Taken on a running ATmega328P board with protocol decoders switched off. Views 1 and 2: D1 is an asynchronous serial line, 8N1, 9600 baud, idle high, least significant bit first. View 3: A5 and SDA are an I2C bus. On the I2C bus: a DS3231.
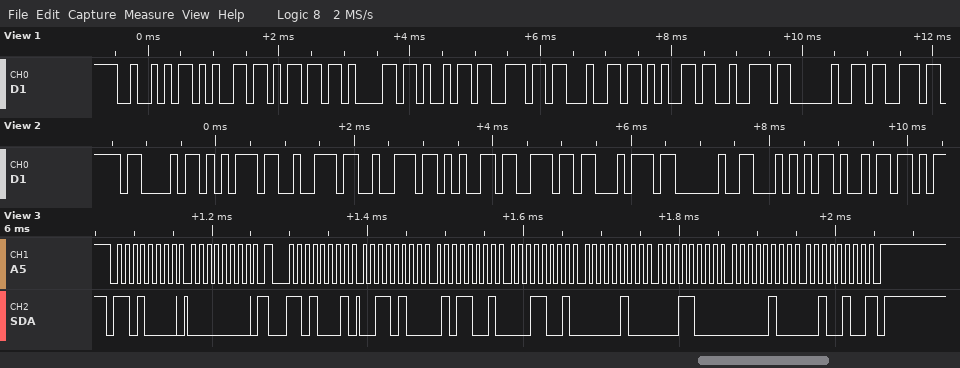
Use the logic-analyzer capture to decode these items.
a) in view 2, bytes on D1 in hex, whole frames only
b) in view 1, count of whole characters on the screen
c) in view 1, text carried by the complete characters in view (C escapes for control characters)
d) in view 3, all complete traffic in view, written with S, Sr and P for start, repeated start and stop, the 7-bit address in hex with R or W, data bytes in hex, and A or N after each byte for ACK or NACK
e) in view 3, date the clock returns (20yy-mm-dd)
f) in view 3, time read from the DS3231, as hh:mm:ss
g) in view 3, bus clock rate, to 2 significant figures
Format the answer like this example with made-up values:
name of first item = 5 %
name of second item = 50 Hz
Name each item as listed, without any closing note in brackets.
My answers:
in view 2, bytes on D1 in hex, whole frames only = 0x43 0x75 0x72 0x72 0x65 0x6E 0x74 0x20 0x54 0x69
in view 1, count of whole characters on the screen = 11
in view 1, text carried by the complete characters in view = "Remainder s"
in view 3, all complete traffic in view, written with S, Sr and P for start, repeated start and stop, the 7-bit address in hex with R or W, data bytes in hex, and A or N after each byte for ACK or NACK = S 68W A 00 A Sr 68R A 34 A 59 A 19 A 04 A 18 A 04 A 24 N P
in view 3, date the clock returns = 2024-04-18
in view 3, time read from the DS3231, as hh:mm:ss = 19:59:34
in view 3, bus clock rate, to 2 significant figures = 100 kHz
